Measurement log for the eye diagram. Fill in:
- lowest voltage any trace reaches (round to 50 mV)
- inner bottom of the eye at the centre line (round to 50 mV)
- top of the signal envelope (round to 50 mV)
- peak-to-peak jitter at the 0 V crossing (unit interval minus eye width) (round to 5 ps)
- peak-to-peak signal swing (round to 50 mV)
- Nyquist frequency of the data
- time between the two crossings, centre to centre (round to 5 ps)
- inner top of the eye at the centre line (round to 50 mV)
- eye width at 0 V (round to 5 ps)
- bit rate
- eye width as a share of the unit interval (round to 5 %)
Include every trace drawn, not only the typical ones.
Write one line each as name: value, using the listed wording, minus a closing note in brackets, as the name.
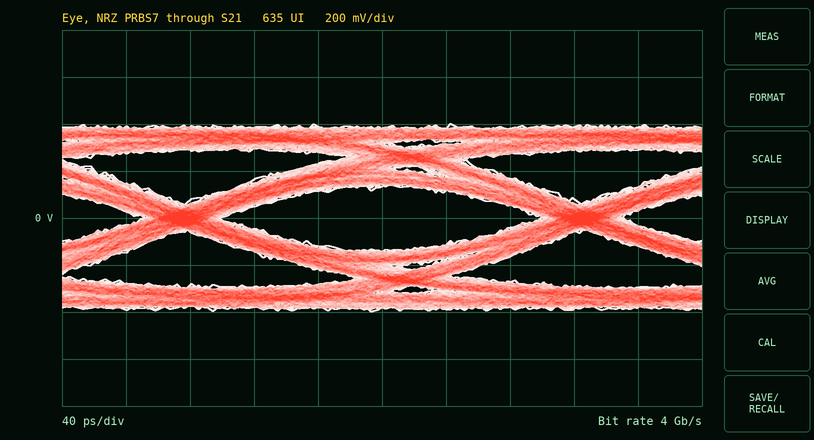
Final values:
lowest voltage any trace reaches: -400 mV
inner bottom of the eye at the centre line: -150 mV
top of the signal envelope: 400 mV
peak-to-peak jitter at the 0 V crossing (unit interval minus eye width): 50 ps
peak-to-peak signal swing: 800 mV
Nyquist frequency of the data: 2 GHz
time between the two crossings, centre to centre: 250 ps
inner top of the eye at the centre line: 150 mV
eye width at 0 V: 200 ps
bit rate: 4 Gb/s
eye width as a share of the unit interval: 80 %
